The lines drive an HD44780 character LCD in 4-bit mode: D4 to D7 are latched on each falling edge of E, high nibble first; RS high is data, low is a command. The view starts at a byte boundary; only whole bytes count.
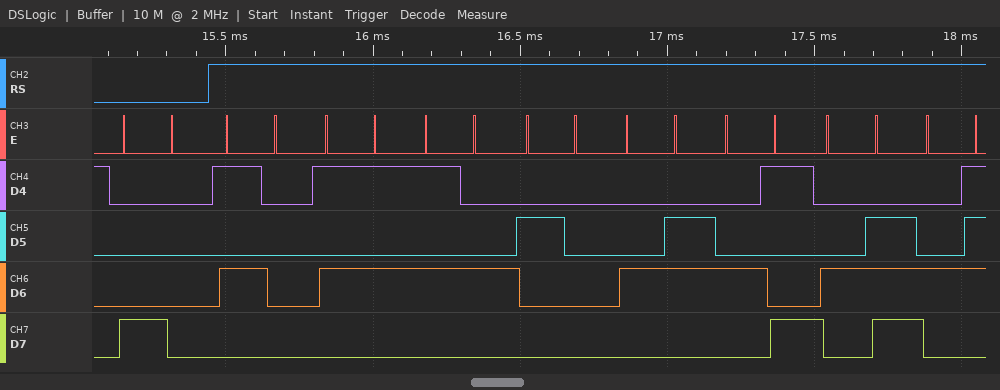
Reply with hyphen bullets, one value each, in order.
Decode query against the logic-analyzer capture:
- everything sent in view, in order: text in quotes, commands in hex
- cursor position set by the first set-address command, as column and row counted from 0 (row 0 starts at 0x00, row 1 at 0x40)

- 0x80 "PUT FING"
- column 0, row 0
